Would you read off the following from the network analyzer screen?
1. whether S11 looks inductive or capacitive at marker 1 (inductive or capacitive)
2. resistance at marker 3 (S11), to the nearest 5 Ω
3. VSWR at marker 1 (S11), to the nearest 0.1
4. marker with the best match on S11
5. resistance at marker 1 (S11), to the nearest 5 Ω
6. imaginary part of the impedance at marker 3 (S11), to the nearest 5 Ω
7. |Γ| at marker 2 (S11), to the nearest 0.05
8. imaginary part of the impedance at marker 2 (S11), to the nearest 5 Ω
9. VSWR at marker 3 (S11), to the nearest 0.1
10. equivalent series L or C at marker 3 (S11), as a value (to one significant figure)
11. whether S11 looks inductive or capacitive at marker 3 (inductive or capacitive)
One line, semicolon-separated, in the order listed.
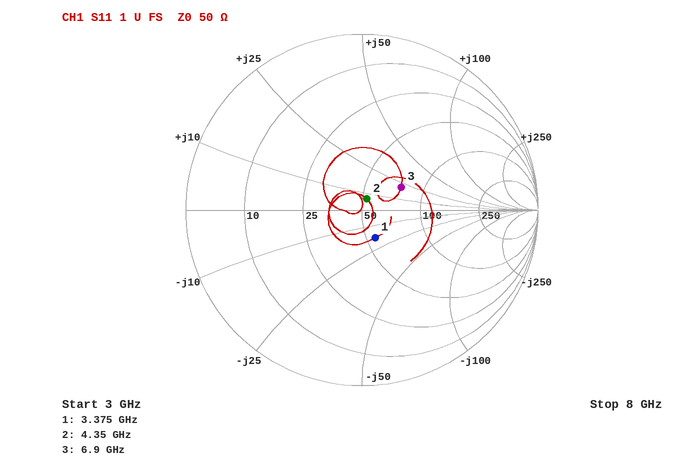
capacitive; 75 Ω; 1.4; marker 2; 55 Ω; +20 Ω; 0.05; +5 Ω; 1.7; 500 pH; inductive
